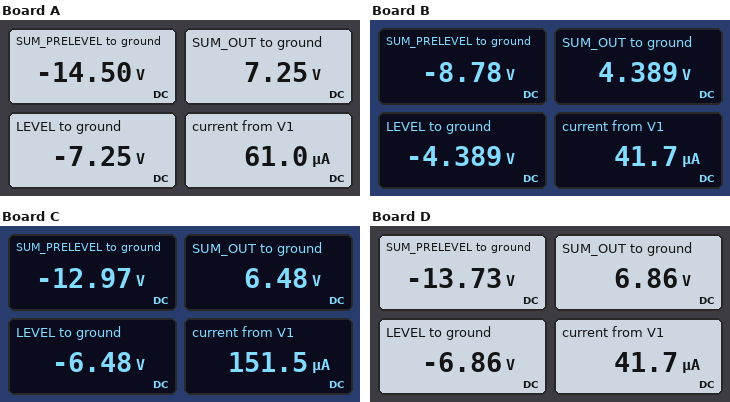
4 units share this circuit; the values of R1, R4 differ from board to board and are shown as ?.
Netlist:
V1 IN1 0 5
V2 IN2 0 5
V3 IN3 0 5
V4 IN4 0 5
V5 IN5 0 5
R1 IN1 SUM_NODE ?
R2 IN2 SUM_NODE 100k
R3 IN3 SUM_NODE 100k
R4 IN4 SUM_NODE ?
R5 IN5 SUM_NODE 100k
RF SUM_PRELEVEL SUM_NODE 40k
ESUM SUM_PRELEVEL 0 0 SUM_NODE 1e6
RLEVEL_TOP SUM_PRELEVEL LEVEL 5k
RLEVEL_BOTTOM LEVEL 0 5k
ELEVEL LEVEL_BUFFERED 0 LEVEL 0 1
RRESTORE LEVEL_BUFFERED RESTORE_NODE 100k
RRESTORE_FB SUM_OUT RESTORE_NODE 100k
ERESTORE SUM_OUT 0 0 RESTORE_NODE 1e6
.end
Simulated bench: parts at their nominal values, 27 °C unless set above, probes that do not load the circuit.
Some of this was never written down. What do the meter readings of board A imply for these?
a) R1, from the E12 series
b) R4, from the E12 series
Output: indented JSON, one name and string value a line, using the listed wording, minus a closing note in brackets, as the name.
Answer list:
{
  "R1, from the E12 series": "82 kΩ",
  "R4, from the E12 series": "33 kΩ"
}
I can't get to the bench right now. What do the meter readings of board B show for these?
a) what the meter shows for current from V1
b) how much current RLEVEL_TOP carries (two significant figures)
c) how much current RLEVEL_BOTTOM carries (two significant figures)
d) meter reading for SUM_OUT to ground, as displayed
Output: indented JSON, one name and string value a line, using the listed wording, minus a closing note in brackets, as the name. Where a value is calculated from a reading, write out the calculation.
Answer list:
{
  "what the meter shows for current from V1": "41.7 µA",
  "how much current RLEVEL_TOP carries": "(-4.389 V - (-8.78 V)) / 5 kΩ = 880 µA",
  "how much current RLEVEL_BOTTOM carries": "(0 V - (-4.389 V)) / 5 kΩ = 880 µA",
  "meter reading for SUM_OUT to ground, as displayed": "4.389 V"
}
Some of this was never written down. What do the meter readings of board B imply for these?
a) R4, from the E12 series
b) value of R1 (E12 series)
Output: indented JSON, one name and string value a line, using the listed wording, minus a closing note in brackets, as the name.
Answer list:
{
  "R4, from the E12 series": "180 kΩ",
  "value of R1": "120 kΩ"
}
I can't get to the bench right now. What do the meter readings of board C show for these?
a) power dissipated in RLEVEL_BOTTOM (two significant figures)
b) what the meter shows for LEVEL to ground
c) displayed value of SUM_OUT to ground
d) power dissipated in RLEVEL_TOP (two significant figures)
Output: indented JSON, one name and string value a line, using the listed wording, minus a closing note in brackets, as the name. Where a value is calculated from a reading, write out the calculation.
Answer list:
{
  "power dissipated in RLEVEL_BOTTOM": "(0 V - (-6.48 V))^2 / 5 kΩ = 8.4 mW",
  "what the meter shows for LEVEL to ground": "-6.48 V",
  "displayed value of SUM_OUT to ground": "6.48 V",
  "power dissipated in RLEVEL_TOP": "(-6.48 V - (-12.97 V))^2 / 5 kΩ = 8.4 mW"
}
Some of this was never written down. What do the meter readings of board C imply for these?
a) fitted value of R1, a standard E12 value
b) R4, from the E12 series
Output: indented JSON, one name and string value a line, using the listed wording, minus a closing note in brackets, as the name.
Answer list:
{
  "fitted value of R1, a standard E12 value": "33 kΩ",
  "R4, from the E12 series": "220 kΩ"
}
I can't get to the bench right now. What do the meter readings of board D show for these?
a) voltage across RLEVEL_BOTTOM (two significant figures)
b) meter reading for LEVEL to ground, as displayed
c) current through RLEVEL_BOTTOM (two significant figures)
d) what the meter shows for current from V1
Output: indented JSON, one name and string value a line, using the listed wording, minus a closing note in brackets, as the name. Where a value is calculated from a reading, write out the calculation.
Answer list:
{
  "voltage across RLEVEL_BOTTOM": "0 V - (-6.86 V) = 6.9 V",
  "meter reading for LEVEL to ground, as displayed": "-6.86 V",
  "current through RLEVEL_BOTTOM": "(0 V - (-6.86 V)) / 5 kΩ = 1.4 mA",
  "what the meter shows for current from V1": "41.7 µA"
}
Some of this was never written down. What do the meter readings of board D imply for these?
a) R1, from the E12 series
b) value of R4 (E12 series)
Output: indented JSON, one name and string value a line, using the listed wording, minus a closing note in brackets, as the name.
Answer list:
{
  "R1, from the E12 series": "120 kΩ",
  "value of R4": "33 kΩ"
}
